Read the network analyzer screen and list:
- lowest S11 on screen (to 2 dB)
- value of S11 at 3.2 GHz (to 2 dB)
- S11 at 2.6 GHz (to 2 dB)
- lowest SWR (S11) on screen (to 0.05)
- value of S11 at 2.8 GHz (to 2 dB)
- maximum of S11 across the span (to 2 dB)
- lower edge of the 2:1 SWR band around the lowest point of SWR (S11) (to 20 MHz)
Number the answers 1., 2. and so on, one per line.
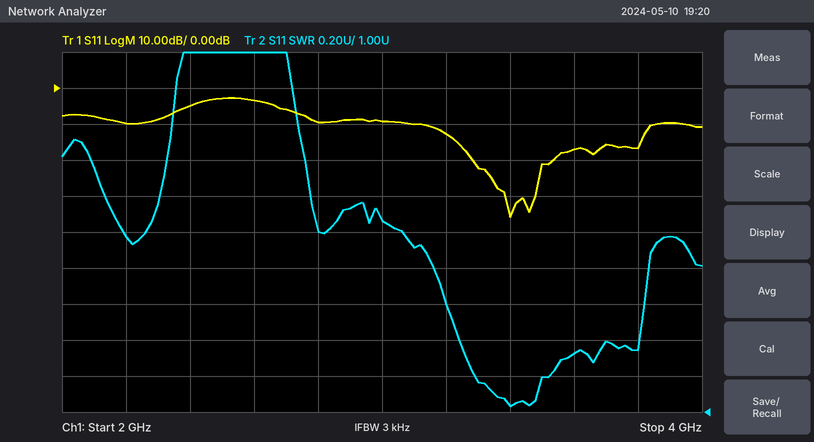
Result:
1. -36 dB
2. -12 dB
3. -4 dB
4. 1.05
5. -10 dB
6. -2 dB
7. 3.06 GHz
